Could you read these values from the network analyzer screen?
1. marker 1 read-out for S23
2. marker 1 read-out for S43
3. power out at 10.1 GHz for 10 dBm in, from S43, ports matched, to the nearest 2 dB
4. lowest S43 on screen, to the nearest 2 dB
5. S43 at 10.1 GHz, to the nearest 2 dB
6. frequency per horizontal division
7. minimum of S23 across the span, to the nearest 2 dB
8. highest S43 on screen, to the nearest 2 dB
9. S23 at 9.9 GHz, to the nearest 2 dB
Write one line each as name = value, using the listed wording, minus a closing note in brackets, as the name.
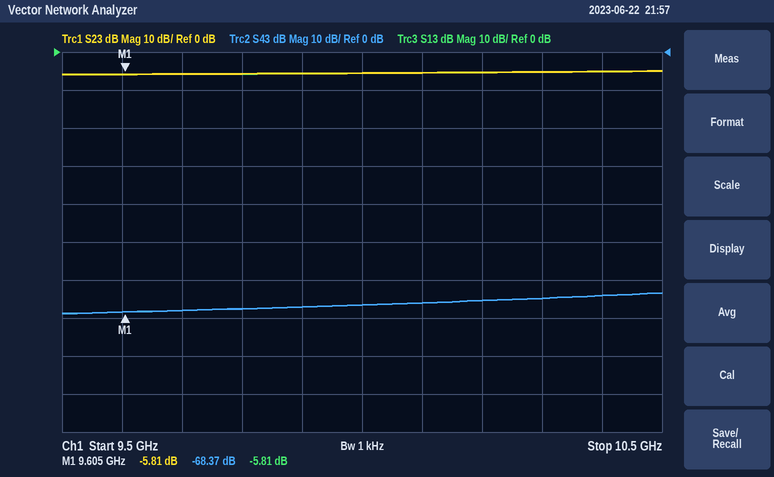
marker 1 read-out for S23 = -5.81 dB
marker 1 read-out for S43 = -68.37 dB
power out at 10.1 GHz for 10 dBm in, from S43, ports matched, to the nearest 2 dB = -56 dBm
lowest S43 on screen, to the nearest 2 dB = -68 dB
S43 at 10.1 GHz, to the nearest 2 dB = -66 dB
frequency per horizontal division = 100 MHz
minimum of S23 across the span, to the nearest 2 dB = -6 dB
highest S43 on screen, to the nearest 2 dB = -64 dB
S23 at 9.9 GHz, to the nearest 2 dB = -6 dB
